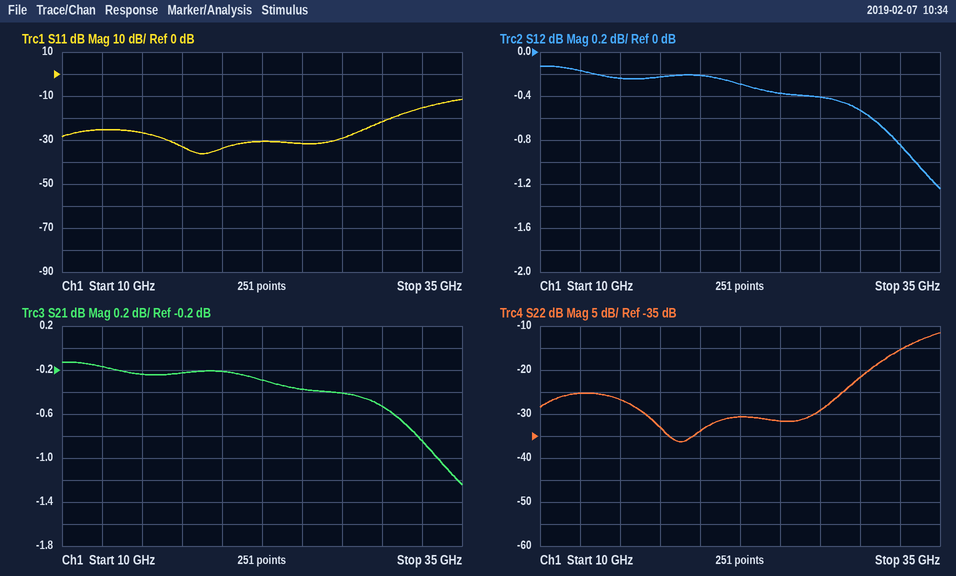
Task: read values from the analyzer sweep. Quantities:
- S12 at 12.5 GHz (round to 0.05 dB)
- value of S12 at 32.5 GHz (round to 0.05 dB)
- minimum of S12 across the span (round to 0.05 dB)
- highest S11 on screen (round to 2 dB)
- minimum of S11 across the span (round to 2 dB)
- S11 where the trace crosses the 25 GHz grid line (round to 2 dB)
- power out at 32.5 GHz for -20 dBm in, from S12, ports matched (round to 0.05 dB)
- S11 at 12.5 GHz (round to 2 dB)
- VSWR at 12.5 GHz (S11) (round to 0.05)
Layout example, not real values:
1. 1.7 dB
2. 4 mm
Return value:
1. -0.15 dB
2. -0.85 dB
3. -1.25 dB
4. -12 dB
5. -36 dB
6. -32 dB
7. -20.85 dBm
8. -26 dB
9. 1.10
